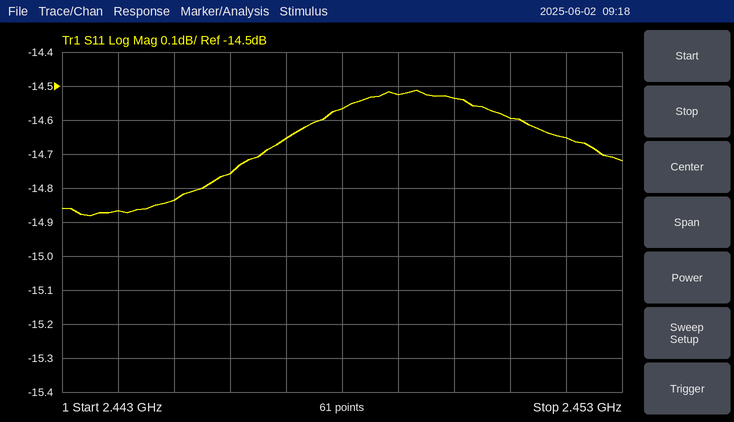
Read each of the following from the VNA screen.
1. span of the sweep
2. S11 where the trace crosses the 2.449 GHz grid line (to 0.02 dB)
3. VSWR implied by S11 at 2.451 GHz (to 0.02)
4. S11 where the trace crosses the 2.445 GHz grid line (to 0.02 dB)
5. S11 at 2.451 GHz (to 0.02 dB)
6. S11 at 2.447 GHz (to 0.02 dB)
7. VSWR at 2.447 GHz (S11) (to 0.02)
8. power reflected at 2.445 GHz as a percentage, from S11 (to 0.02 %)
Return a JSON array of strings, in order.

["10 MHz", "-14.52 dB", "1.46", "-14.84 dB", "-14.60 dB", "-14.66 dB", "1.46", "3.28 %"]
